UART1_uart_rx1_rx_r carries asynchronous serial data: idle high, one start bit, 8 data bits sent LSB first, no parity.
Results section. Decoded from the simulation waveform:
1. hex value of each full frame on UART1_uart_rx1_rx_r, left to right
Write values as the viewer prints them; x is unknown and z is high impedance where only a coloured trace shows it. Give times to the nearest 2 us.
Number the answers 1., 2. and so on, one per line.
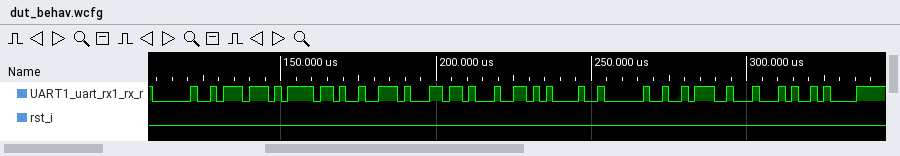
1. 20, 77, 6F, 72, 6C, 64, 21, 20, 3A, 44, 0A
